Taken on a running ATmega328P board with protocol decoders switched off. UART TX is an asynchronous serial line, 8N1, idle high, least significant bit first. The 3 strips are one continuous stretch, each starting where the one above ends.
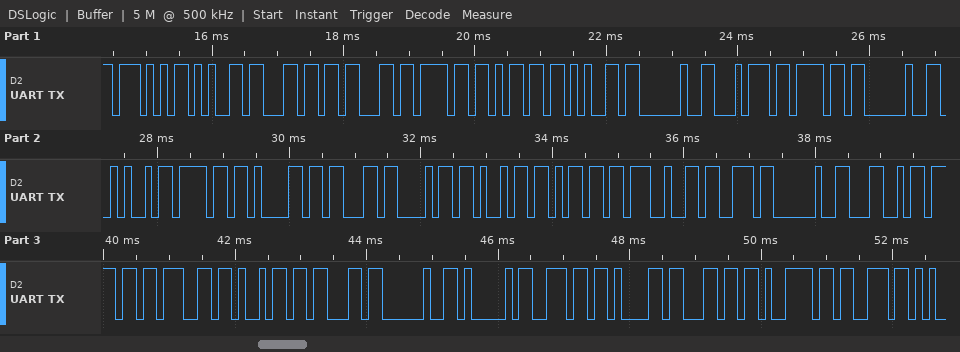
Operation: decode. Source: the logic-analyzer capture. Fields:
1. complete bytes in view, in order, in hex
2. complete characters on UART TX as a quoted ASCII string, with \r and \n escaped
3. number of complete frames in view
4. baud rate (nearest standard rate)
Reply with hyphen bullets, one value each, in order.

- 57 65 6C 63 6F 6D 65 20 74 6F 20 4A 6F 61 63 68 69 6D 27 73 20 4C 6F 67 69 63 20 41 6E 61 6C 79 73
- "Welcome to Joachim's Logic Analys"
- 33
- 9600 baud
